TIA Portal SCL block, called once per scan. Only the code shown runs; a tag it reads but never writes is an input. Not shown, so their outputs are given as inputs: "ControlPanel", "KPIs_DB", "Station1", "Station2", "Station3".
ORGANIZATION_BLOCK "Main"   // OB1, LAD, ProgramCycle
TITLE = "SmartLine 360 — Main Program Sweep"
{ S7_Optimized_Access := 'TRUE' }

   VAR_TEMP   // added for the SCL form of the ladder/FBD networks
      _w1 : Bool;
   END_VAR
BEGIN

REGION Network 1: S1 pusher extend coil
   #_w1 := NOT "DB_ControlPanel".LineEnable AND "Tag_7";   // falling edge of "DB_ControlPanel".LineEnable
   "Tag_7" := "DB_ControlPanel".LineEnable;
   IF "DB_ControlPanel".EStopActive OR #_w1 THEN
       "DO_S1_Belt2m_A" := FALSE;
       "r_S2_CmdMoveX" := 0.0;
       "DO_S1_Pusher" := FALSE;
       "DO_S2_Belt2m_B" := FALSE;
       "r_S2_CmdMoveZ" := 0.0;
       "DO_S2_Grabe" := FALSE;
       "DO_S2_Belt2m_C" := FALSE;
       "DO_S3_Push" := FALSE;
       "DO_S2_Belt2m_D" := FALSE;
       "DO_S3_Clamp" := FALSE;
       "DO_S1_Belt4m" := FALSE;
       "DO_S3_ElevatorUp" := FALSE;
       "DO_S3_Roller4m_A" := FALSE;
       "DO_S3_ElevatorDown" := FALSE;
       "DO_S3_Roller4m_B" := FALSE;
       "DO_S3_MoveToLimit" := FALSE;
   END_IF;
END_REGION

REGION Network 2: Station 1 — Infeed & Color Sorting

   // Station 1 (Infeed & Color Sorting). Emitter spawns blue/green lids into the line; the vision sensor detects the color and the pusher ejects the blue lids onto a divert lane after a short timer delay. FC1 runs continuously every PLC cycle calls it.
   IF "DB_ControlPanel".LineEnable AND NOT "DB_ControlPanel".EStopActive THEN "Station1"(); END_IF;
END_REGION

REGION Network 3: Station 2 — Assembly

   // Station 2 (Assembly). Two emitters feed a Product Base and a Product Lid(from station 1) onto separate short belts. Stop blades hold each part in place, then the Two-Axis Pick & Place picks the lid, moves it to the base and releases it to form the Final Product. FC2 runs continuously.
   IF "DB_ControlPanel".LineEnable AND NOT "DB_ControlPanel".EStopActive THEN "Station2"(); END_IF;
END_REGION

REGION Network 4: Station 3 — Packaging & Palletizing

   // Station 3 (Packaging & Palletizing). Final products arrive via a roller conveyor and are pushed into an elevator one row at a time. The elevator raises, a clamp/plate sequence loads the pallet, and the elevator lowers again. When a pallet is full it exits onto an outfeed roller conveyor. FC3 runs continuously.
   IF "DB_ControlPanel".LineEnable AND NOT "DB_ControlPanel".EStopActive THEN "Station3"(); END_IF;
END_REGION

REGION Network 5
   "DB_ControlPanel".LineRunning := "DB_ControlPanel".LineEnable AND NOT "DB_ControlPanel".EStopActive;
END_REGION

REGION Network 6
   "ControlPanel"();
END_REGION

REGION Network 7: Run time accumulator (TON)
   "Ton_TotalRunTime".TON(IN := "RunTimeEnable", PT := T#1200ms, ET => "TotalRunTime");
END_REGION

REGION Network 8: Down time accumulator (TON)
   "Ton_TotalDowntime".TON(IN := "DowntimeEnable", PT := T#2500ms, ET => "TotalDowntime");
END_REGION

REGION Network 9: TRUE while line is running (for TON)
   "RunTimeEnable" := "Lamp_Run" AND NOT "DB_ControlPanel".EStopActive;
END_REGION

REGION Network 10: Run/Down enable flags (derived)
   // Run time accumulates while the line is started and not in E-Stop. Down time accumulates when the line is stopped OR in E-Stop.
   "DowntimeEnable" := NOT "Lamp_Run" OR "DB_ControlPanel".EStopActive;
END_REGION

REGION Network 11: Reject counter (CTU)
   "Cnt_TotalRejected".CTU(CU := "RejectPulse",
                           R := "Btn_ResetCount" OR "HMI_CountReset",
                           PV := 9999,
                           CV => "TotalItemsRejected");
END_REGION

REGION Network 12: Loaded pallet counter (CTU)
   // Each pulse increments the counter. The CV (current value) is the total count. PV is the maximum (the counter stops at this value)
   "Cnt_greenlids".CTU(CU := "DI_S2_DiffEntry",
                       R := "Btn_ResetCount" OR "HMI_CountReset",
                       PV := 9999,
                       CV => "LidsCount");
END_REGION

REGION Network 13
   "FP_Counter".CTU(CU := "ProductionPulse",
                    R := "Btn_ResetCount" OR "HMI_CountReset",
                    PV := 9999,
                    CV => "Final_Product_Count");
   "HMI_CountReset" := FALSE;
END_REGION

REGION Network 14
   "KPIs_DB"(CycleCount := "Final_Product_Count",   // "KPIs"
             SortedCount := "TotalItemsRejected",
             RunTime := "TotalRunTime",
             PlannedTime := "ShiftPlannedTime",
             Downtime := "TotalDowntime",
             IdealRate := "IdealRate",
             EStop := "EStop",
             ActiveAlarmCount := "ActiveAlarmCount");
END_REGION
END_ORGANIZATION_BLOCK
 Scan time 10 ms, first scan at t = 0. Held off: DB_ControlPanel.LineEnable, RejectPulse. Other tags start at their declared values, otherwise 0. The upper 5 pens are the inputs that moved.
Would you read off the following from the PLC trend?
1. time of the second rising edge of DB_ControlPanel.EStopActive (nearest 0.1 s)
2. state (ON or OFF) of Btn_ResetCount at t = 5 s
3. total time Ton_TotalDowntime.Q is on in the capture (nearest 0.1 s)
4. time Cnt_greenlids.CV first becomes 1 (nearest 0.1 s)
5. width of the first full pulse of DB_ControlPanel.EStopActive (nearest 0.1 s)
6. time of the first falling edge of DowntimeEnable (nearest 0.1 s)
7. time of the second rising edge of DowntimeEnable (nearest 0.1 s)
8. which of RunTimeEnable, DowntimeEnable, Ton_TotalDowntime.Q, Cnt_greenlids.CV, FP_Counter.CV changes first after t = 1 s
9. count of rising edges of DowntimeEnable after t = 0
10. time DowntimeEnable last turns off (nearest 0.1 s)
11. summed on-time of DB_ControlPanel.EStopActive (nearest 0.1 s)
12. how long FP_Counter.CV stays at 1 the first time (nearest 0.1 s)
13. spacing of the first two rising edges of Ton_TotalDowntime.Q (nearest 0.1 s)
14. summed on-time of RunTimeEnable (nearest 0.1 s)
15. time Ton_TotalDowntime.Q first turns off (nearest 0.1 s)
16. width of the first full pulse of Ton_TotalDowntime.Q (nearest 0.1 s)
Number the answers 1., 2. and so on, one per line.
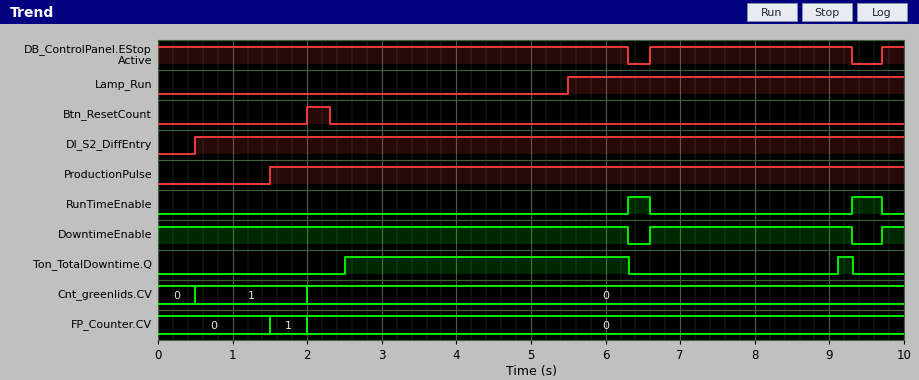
1. 9.7 s
2. OFF
3. 4.0 s
4. 0.5 s
5. 2.7 s
6. 6.3 s
7. 9.7 s
8. FP_Counter.CV
9. 2
10. 9.3 s
11. 9.3 s
12. 0.5 s
13. 6.6 s
14. 0.7 s
15. 6.3 s
16. 3.8 s
